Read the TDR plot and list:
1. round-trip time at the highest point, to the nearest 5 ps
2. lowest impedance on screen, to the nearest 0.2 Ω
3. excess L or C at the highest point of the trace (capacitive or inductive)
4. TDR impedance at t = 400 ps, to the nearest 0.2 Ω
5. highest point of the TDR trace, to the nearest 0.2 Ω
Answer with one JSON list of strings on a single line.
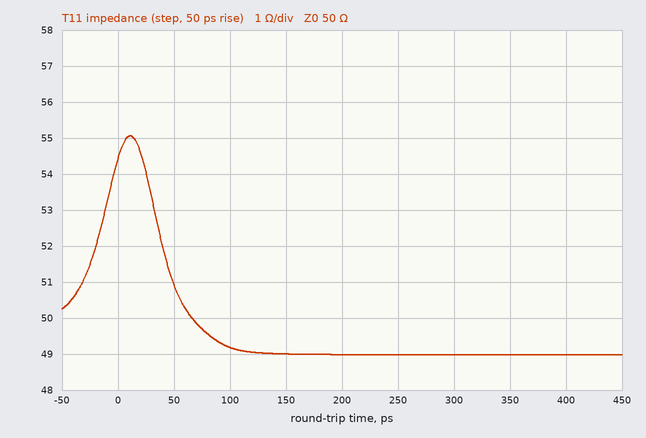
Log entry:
["10 ps", "49.0 Ω", "inductive", "49.0 Ω", "55.0 Ω"]
